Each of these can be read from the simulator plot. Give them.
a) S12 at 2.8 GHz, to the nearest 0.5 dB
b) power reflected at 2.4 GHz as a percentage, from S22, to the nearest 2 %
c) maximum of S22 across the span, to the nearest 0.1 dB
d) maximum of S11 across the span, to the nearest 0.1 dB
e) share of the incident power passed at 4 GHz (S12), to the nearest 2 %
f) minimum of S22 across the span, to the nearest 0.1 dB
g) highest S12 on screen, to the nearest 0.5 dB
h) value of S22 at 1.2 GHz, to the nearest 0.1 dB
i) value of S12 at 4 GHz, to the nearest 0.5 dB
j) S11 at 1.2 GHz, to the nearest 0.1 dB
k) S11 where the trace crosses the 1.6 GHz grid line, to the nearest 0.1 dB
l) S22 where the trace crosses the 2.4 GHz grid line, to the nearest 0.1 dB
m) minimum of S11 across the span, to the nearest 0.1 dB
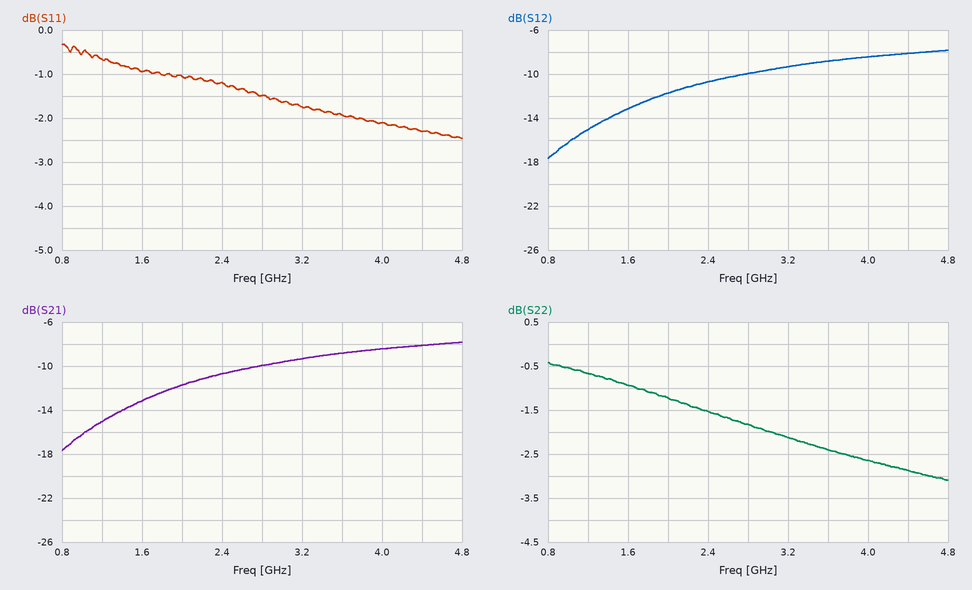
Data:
-10.0 dB
70 %
-0.4 dB
-0.3 dB
14 %
-3.1 dB
-8.0 dB
-0.7 dB
-8.5 dB
-0.7 dB
-0.9 dB
-1.5 dB
-2.5 dB
